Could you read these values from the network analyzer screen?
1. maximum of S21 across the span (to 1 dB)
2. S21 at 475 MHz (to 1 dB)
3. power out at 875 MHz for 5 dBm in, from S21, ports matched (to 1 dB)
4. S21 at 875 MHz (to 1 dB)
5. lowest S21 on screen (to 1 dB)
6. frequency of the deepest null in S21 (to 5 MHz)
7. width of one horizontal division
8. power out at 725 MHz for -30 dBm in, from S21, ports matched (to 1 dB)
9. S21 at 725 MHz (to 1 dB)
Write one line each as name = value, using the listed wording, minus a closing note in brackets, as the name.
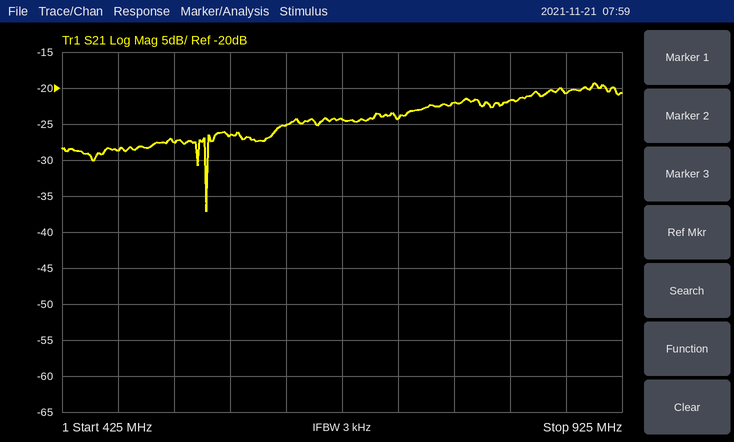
maximum of S21 across the span = -19 dB
S21 at 475 MHz = -29 dB
power out at 875 MHz for 5 dBm in, from S21, ports matched = -16 dBm
S21 at 875 MHz = -21 dB
lowest S21 on screen = -37 dB
frequency of the deepest null in S21 = 555 MHz
width of one horizontal division = 50 MHz
power out at 725 MHz for -30 dBm in, from S21, ports matched = -54 dBm
S21 at 725 MHz = -24 dB
